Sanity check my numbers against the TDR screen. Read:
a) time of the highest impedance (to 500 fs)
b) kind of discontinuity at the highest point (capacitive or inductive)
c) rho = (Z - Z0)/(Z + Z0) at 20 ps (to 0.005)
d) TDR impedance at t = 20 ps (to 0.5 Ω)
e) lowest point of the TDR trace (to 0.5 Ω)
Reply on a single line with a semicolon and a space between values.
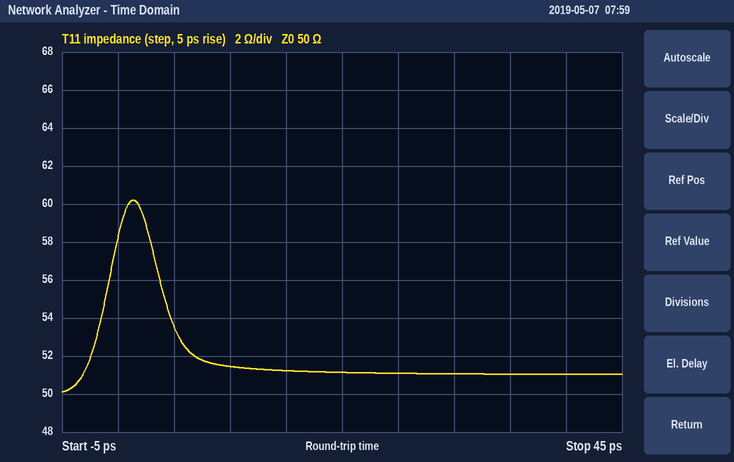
1.5 ps; inductive; +0.010; 51.0 Ω; 50.0 Ω
